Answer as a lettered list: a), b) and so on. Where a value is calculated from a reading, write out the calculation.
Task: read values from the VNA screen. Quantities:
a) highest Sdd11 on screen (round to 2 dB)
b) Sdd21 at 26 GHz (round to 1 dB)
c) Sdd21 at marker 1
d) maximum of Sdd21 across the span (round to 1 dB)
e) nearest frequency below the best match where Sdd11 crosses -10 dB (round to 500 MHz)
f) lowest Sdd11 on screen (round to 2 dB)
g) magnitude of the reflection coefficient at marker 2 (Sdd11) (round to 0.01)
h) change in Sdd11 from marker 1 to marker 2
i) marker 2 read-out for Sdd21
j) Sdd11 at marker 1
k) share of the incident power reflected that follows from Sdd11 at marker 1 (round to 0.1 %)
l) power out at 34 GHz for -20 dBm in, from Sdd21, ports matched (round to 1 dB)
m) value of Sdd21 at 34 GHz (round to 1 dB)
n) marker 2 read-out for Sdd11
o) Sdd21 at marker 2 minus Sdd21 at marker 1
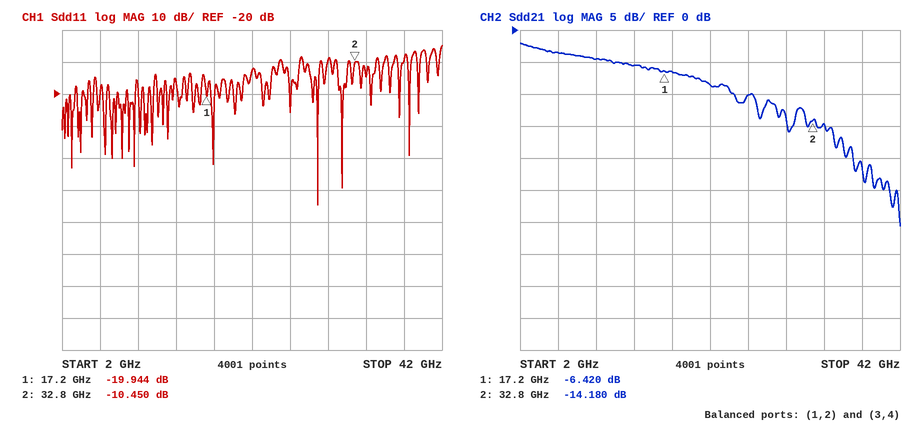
a) -4 dB
b) -10 dB
c) -6.420 dB
d) -2 dB
e) 27.5 GHz
f) -54 dB
g) 10^(-10.45/20) ≈ 0.30
h) -10.45 − (-19.944) = 9.494 dB
i) -14.180 dB
j) -19.944 dB
k) 10^(-19.944/10) ≈ 1.0 %
l) -20 dBm + (-15 dB) = -35 dBm
m) -15 dB
n) -10.450 dB
o) -14.18 − (-6.42) = -7.760 dB
